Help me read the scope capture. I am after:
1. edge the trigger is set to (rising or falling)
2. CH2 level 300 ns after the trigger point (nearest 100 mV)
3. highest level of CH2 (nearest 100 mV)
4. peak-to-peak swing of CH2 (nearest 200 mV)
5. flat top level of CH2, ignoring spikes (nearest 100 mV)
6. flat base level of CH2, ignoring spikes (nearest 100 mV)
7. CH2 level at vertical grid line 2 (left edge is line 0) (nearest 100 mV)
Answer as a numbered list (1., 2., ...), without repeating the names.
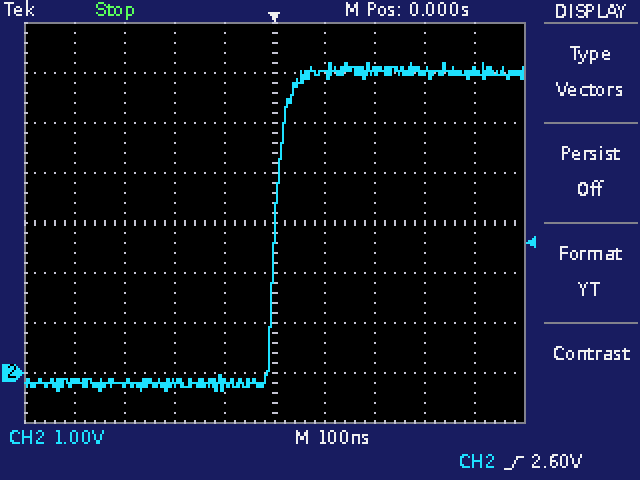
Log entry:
1. rising
2. 6.0 V
3. 6.2 V
4. 6.6 V
5. 6.0 V
6. -200 mV
7. -200 mV
